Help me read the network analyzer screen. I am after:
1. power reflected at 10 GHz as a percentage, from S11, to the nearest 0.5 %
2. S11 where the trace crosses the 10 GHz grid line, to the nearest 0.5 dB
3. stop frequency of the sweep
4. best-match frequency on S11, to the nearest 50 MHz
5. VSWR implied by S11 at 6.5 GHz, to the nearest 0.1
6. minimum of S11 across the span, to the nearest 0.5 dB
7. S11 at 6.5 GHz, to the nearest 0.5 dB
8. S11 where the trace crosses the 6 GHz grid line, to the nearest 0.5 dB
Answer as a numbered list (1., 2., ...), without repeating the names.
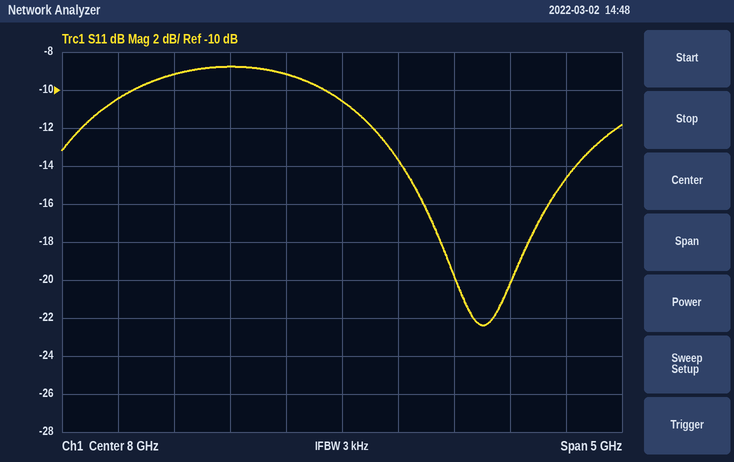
1. 3.5 %
2. -14.5 dB
3. 10.5 GHz
4. 9.25 GHz
5. 2.1
6. -22.5 dB
7. -9.0 dB
8. -10.5 dB
